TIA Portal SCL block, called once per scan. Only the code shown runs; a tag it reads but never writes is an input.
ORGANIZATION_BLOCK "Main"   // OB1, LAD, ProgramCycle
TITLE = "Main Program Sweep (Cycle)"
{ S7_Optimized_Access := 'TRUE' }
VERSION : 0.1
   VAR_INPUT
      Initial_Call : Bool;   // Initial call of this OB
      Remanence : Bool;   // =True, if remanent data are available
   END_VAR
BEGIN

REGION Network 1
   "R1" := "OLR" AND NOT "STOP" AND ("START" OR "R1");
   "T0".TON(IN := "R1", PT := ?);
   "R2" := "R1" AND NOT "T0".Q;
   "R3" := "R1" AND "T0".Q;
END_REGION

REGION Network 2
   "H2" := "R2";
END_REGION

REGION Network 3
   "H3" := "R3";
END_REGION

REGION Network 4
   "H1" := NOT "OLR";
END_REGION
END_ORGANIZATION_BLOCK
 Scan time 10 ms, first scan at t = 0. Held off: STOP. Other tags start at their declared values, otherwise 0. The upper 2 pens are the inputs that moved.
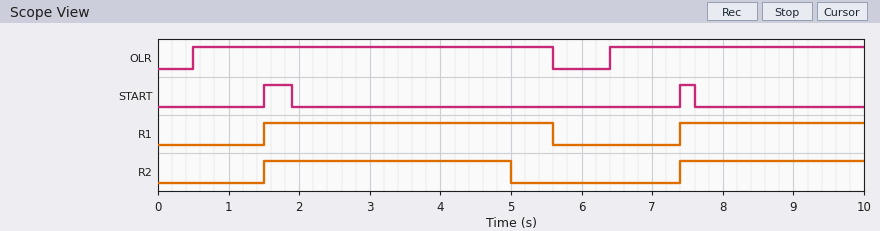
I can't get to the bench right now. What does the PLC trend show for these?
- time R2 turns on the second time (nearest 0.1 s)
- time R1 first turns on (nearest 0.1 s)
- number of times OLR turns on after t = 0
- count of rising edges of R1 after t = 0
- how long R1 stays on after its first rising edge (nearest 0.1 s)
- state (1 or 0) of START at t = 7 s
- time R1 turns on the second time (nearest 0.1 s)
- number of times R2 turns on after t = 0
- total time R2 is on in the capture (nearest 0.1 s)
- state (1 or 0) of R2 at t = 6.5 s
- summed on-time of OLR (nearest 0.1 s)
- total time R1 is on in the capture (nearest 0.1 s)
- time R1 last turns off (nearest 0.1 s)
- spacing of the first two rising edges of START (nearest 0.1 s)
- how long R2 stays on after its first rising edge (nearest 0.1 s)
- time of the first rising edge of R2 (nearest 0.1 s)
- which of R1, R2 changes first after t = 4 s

7.4 s
1.5 s
2
2
4.1 s
0
7.4 s
2
6.1 s
0
8.7 s
6.7 s
5.6 s
5.9 s
3.5 s
1.5 s
R2
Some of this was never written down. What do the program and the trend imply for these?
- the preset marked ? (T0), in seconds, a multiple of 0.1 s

3.5 s
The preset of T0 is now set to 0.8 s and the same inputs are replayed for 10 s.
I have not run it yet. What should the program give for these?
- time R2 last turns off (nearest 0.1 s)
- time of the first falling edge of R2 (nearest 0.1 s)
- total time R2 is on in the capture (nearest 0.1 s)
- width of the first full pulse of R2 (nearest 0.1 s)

8.2 s
2.3 s
1.6 s
0.8 s
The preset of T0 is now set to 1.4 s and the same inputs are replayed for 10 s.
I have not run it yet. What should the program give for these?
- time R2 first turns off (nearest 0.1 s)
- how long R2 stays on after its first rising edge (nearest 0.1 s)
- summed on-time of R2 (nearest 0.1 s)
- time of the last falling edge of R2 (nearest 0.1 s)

2.9 s
1.4 s
2.8 s
8.8 s
